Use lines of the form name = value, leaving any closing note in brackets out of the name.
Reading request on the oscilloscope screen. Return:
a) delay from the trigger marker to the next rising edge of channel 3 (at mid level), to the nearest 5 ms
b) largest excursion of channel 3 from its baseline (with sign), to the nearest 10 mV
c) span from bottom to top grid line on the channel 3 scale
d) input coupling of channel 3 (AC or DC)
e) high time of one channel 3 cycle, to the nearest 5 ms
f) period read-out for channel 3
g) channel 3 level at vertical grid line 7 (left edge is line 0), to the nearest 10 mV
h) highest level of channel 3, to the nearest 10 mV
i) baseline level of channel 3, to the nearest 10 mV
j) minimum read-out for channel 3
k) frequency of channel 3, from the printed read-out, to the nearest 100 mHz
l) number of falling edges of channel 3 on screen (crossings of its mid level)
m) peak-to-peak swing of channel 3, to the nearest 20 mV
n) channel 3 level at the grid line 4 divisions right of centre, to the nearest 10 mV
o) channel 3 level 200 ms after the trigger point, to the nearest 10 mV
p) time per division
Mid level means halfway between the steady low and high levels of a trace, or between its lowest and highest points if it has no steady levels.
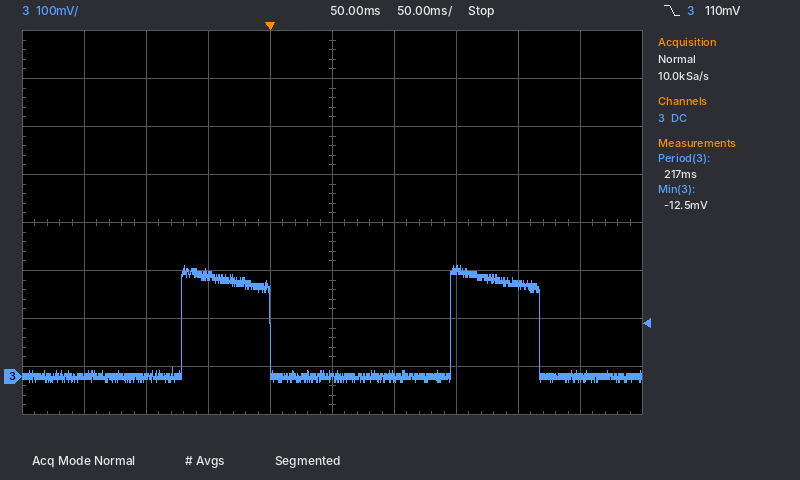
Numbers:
delay from the trigger marker to the next rising edge of channel 3 (at mid level), to the nearest 5 ms = 145 ms
largest excursion of channel 3 from its baseline (with sign), to the nearest 10 mV = +230 mV
span from bottom to top grid line on the channel 3 scale = 800 mV
input coupling of channel 3 = DC
high time of one channel 3 cycle, to the nearest 5 ms = 70 ms
period read-out for channel 3 = 217 ms
channel 3 level at vertical grid line 7 (left edge is line 0), to the nearest 10 mV = 220 mV
highest level of channel 3, to the nearest 10 mV = 230 mV
baseline level of channel 3, to the nearest 10 mV = 0 mV
minimum read-out for channel 3 = -12.5 mV
frequency of channel 3, from the printed read-out, to the nearest 100 mHz = 4.6 Hz
number of falling edges of channel 3 on screen = 2
peak-to-peak swing of channel 3, to the nearest 20 mV = 240 mV
channel 3 level at the grid line 4 divisions right of centre, to the nearest 10 mV = 0 mV
channel 3 level 200 ms after the trigger point, to the nearest 10 mV = 190 mV
time per division = 50 ms
